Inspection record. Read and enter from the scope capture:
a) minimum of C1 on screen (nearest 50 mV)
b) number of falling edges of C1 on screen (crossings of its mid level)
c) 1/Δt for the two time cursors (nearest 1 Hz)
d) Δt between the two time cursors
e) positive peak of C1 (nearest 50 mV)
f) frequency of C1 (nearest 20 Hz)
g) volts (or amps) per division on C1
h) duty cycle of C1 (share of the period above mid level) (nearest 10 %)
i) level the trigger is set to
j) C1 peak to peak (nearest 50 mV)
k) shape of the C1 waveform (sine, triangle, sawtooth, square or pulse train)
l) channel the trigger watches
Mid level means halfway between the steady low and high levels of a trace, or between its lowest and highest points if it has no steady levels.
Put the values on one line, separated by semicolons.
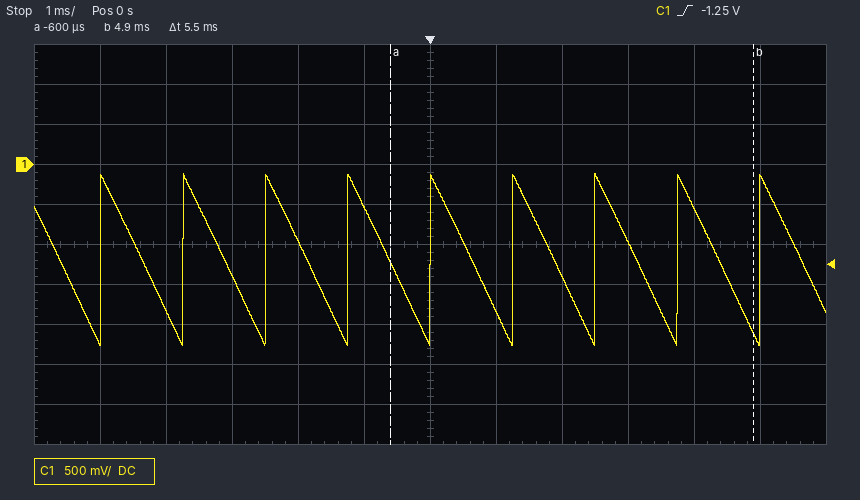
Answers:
-2.25 V; 10; 182 Hz; 5.5 ms; -100 mV; 800 Hz; 500 mV; 50 %; -1.25 V; 2.15 V; sawtooth; C1
